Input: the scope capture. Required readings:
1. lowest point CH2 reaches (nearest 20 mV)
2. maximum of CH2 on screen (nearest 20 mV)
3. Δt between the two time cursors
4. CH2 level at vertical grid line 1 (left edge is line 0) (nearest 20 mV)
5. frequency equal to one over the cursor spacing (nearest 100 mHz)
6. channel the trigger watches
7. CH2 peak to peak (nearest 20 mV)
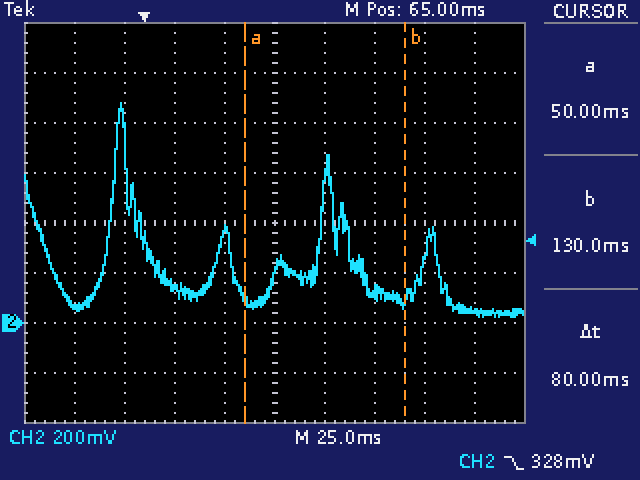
20 mV
880 mV
80 ms
60 mV
12.5 Hz
CH2
860 mV
